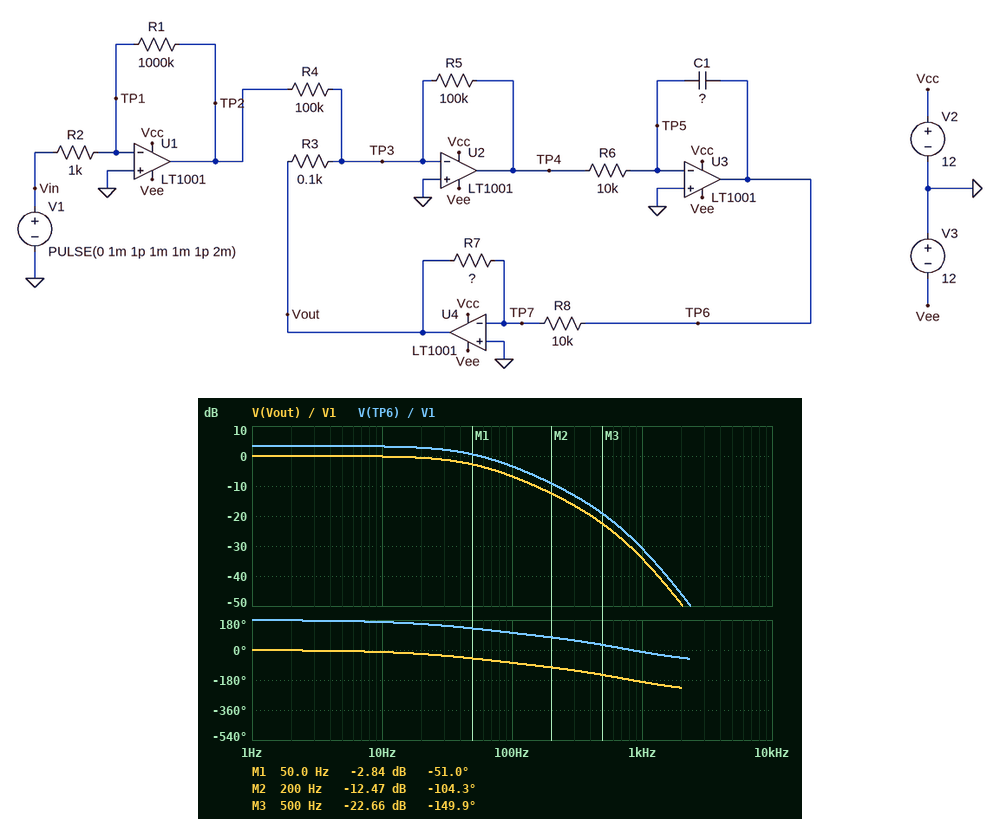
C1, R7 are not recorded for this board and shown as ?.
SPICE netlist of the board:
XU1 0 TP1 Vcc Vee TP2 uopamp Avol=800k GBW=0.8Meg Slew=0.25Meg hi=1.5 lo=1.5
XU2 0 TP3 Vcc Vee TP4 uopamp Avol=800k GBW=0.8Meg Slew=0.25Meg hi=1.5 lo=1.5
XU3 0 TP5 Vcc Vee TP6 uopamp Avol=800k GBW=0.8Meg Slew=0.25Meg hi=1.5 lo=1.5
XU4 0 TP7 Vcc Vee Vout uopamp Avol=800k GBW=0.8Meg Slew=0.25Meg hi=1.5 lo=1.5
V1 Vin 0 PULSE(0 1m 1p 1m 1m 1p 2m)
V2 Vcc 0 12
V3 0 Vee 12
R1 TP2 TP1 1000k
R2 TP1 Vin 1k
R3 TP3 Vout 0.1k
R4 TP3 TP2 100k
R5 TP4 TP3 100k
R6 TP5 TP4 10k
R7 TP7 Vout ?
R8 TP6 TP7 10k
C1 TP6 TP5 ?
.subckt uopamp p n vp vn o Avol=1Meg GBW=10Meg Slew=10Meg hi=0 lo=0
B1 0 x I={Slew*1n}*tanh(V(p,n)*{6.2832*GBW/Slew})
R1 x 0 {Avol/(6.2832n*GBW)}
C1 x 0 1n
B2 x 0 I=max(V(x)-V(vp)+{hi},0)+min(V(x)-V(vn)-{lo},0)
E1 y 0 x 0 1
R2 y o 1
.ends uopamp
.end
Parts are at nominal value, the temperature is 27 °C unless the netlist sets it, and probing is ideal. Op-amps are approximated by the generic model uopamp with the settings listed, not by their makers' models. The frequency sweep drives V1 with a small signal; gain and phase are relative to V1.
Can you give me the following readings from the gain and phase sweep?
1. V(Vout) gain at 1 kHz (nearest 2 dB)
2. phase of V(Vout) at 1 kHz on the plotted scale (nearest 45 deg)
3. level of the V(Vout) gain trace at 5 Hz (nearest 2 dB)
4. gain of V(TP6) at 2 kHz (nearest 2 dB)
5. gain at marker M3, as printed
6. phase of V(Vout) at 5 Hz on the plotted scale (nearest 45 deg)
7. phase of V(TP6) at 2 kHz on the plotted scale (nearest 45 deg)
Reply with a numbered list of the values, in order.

1. -34 dB
2. -180 deg
3. 0 dB
4. -46 dB
5. -22.66 dB
6. 0 deg
7. -45 deg
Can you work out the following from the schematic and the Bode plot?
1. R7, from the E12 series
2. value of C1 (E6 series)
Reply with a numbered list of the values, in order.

1. 6.8 kΩ
2. 220 µF
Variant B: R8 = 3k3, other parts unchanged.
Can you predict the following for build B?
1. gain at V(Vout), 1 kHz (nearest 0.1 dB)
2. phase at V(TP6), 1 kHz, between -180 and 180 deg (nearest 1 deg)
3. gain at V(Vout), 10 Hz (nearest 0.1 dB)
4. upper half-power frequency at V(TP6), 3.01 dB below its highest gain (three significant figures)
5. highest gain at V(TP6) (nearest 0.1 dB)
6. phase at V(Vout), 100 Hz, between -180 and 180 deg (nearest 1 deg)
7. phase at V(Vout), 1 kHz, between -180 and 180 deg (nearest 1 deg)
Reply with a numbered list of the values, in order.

1. -24.1 dB
2. -9 deg
3. 0 dB
4. 173 Hz
5. -6.3 dB
6. -43 deg
7. 171 deg
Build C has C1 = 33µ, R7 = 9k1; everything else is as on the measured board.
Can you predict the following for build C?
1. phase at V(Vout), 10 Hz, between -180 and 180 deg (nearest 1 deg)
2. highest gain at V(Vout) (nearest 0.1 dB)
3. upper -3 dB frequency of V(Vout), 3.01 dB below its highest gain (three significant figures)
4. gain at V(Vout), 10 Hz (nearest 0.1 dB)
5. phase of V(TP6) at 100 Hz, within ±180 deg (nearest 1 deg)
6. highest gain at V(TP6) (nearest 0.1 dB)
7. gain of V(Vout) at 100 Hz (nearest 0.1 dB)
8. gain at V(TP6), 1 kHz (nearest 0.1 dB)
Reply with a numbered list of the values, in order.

1. -2 deg
2. 0 dB
3. 511 Hz
4. 0 dB
5. 160 deg
6. 0.8 dB
7. -0.1 dB
8. -12.6 dB
